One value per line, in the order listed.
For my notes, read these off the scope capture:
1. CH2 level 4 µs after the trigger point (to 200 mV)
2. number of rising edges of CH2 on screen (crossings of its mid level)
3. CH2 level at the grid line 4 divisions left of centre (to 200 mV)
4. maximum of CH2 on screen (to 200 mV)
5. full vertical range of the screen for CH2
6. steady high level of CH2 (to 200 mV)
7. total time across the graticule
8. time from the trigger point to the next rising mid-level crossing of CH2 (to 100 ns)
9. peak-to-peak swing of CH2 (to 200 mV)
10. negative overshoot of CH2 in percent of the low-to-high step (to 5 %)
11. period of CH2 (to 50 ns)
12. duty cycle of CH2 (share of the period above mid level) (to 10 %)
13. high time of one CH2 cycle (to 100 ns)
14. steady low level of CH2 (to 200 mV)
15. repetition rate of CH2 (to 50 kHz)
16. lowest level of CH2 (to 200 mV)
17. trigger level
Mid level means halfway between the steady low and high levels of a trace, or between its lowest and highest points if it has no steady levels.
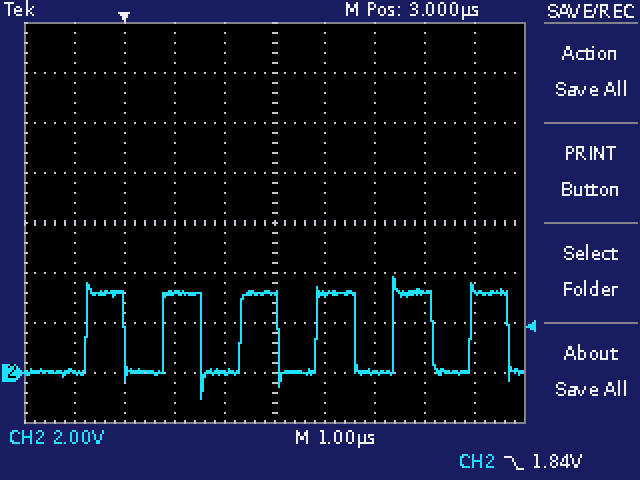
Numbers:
3.2 V
6
0.0 V
3.8 V
16 V
3.2 V
10 µs
800 ns
4.8 V
35 %
1.55 µs
50 %
800 ns
0.0 V
650 kHz
-1.0 V
1.84 V
